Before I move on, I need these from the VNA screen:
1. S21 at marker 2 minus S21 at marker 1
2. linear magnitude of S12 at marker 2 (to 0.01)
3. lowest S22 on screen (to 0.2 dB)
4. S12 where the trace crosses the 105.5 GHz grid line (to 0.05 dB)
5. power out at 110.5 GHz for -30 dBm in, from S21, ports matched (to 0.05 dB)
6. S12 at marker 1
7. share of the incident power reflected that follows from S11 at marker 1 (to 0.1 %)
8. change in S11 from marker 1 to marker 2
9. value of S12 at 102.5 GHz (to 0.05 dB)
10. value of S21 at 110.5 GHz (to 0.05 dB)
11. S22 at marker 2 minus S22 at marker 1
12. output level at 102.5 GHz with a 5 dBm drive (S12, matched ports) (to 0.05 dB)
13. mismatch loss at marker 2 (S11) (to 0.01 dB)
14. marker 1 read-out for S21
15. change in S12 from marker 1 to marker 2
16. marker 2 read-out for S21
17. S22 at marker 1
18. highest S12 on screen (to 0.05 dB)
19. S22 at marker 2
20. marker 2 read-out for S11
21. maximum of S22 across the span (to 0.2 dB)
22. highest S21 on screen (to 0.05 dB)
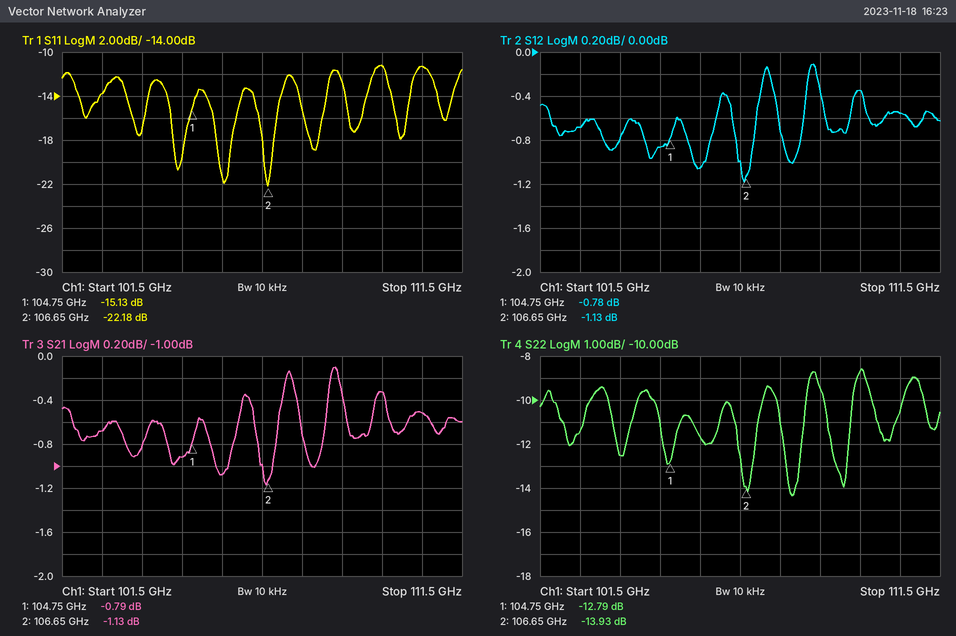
-0.34 dB
0.88
-14.4 dB
-1.05 dB
-30.50 dBm
-0.78 dB
3.1 %
-7.05 dB
-0.70 dB
-0.50 dB
-1.14 dB
4.30 dBm
0.03 dB
-0.79 dB
-0.35 dB
-1.13 dB
-12.79 dB
-0.10 dB
-13.93 dB
-22.18 dB
-8.6 dB
-0.10 dB
